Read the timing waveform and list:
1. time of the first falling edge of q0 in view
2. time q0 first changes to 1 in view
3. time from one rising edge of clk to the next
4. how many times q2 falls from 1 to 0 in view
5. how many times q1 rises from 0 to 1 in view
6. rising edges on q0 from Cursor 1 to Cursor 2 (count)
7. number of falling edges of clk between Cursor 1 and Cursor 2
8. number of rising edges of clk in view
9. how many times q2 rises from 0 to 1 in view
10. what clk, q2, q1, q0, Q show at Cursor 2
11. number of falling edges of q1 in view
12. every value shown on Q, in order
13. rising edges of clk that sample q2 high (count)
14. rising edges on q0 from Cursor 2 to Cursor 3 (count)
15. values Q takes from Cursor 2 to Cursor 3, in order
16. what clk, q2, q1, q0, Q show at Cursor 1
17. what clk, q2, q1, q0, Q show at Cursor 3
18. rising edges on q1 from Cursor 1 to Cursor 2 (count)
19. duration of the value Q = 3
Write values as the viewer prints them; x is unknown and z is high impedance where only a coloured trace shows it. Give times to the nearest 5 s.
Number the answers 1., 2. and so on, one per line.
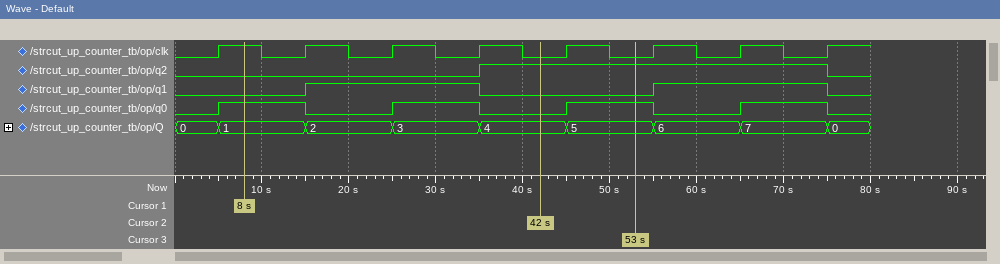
1. 15 s
2. 5 s
3. 10 s
4. 1
5. 2
6. 1
7. 4
8. 8
9. 1
10. clk=0, q2=1, q1=0, q0=0, Q=4
11. 2
12. 0, 1, 2, 3, 4, 5, 6, 7, 0
13. 4
14. 1
15. 4, 5
16. clk=1, q2=0, q1=0, q0=1, Q=1
17. clk=0, q2=1, q1=0, q0=1, Q=5
18. 1
19. 10 s
